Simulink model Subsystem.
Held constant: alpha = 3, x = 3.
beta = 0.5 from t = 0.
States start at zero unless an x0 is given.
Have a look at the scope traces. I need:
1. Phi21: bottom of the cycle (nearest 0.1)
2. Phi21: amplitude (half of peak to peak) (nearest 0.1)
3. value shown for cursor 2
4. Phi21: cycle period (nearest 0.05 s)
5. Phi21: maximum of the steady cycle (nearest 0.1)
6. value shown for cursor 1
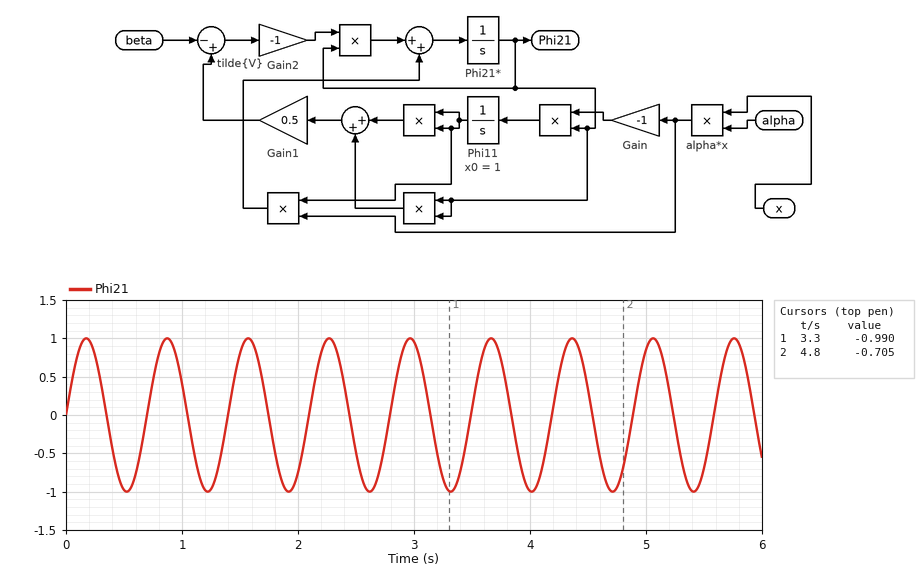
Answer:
-1.0
1.0
-0.705
0.70 s
1.0
-0.990
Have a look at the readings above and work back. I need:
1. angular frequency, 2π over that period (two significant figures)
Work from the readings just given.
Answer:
9.0 rad/s
